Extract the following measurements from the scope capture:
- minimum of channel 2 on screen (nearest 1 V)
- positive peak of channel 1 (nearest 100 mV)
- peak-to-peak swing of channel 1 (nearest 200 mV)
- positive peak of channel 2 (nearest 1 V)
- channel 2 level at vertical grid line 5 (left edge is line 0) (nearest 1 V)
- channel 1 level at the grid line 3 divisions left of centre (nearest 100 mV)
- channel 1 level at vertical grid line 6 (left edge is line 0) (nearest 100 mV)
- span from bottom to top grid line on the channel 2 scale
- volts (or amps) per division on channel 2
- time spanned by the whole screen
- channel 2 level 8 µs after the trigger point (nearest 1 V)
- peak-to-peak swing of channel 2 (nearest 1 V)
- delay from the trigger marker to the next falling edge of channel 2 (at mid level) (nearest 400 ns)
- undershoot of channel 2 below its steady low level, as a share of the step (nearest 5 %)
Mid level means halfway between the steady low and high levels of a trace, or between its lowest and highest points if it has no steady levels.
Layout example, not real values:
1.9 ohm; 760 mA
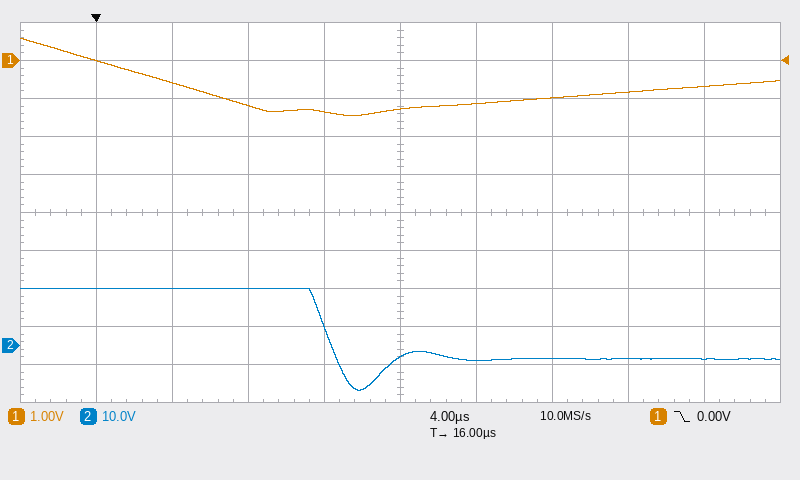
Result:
-12 V; 600 mV; 2.0 V; 15 V; -3 V; -600 mV; -1.1 V; 100 V; 10 V; 40 µs; 15 V; 27 V; 12.0 µs; 45 %
